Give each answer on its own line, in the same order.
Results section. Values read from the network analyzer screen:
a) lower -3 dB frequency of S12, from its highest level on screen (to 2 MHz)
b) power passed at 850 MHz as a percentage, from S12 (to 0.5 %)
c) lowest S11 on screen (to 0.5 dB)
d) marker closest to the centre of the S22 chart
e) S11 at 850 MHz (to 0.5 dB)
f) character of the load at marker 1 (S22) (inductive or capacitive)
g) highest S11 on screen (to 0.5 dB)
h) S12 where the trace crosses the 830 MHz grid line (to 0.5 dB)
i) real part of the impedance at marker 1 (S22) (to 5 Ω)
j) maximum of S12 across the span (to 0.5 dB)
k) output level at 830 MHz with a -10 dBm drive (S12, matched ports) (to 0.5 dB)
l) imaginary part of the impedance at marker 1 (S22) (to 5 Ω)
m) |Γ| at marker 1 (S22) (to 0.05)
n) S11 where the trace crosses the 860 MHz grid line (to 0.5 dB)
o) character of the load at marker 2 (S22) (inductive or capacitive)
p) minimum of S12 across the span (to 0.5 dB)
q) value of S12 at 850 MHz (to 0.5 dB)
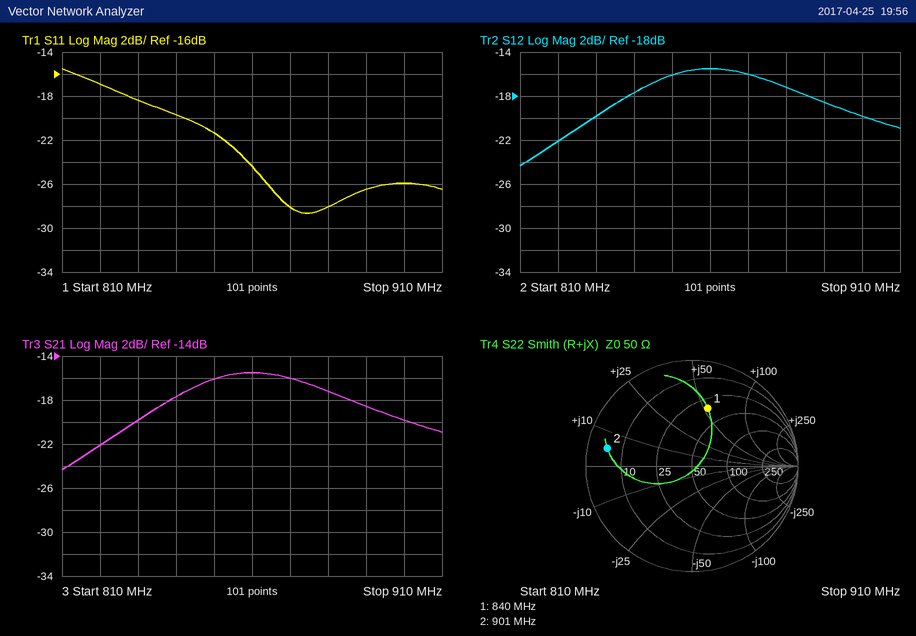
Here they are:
836 MHz
2.5 %
-28.5 dB
marker 1
-21.5 dB
inductive
-15.5 dB
-20.0 dB
35 Ω
-15.5 dB
-30.0 dBm
+55 Ω
0.55
-24.5 dB
inductive
-24.5 dB
-16.0 dB
